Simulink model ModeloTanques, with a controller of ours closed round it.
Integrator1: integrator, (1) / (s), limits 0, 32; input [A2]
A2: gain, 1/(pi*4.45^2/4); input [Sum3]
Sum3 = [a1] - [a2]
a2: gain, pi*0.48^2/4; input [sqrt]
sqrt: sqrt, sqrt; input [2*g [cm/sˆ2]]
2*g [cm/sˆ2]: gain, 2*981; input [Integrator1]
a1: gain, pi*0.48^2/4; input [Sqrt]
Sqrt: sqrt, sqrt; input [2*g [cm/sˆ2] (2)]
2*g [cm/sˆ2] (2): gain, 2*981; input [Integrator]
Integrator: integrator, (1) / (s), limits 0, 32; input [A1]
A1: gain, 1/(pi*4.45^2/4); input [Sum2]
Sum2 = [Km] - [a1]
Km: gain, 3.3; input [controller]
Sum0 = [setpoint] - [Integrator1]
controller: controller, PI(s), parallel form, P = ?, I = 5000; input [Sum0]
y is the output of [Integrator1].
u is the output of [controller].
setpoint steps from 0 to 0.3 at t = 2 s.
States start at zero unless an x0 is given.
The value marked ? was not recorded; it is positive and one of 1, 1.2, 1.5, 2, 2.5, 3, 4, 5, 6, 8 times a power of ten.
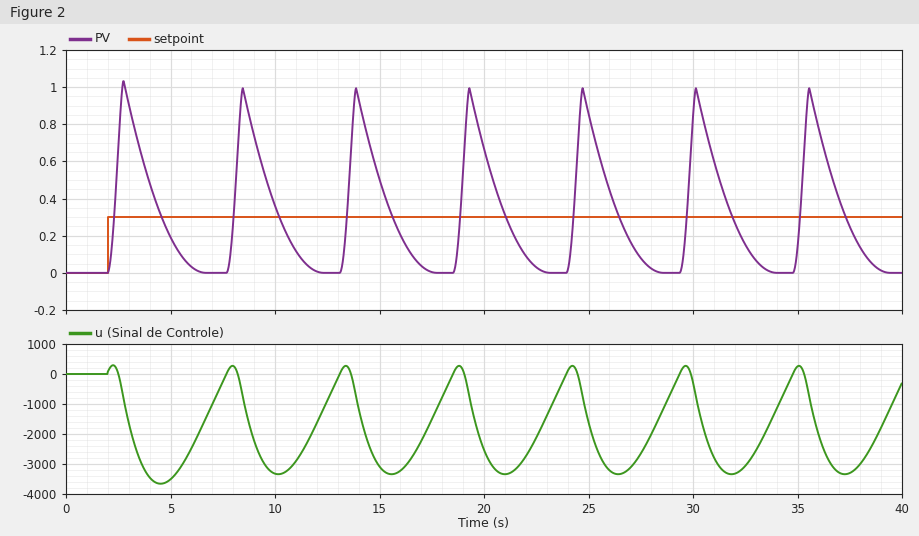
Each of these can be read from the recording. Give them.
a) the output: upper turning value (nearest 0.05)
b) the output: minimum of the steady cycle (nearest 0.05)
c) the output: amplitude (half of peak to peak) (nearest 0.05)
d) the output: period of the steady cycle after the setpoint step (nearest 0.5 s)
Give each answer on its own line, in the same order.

1.00
0.00
0.50
5.5 s
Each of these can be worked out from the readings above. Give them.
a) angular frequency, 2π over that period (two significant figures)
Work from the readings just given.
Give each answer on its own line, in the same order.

1.1 rad/s
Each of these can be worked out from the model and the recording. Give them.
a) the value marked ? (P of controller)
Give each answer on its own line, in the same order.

250
